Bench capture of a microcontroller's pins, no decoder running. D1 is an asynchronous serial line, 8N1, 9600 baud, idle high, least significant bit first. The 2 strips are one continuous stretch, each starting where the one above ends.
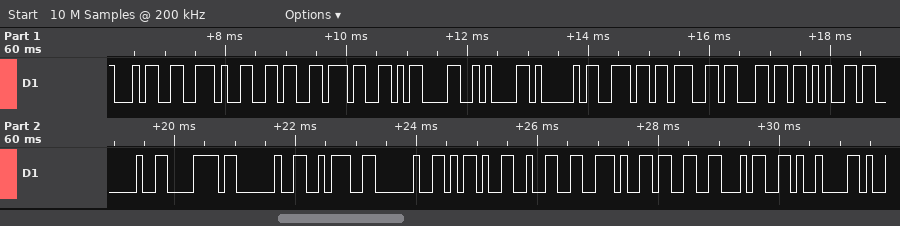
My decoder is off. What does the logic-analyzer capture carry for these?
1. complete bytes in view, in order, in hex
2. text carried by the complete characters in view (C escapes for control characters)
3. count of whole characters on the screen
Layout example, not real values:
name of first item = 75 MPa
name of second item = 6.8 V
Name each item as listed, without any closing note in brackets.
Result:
complete bytes in view, in order, in hex = 34 2E 36 37 0D 0A 41 6E 67 6C 65 20 78 20 3A 20 2D 32 2E 33 34 09
text carried by the complete characters in view = "4.67\r\nAngle x : -2.34\t"
count of whole characters on the screen = 22
